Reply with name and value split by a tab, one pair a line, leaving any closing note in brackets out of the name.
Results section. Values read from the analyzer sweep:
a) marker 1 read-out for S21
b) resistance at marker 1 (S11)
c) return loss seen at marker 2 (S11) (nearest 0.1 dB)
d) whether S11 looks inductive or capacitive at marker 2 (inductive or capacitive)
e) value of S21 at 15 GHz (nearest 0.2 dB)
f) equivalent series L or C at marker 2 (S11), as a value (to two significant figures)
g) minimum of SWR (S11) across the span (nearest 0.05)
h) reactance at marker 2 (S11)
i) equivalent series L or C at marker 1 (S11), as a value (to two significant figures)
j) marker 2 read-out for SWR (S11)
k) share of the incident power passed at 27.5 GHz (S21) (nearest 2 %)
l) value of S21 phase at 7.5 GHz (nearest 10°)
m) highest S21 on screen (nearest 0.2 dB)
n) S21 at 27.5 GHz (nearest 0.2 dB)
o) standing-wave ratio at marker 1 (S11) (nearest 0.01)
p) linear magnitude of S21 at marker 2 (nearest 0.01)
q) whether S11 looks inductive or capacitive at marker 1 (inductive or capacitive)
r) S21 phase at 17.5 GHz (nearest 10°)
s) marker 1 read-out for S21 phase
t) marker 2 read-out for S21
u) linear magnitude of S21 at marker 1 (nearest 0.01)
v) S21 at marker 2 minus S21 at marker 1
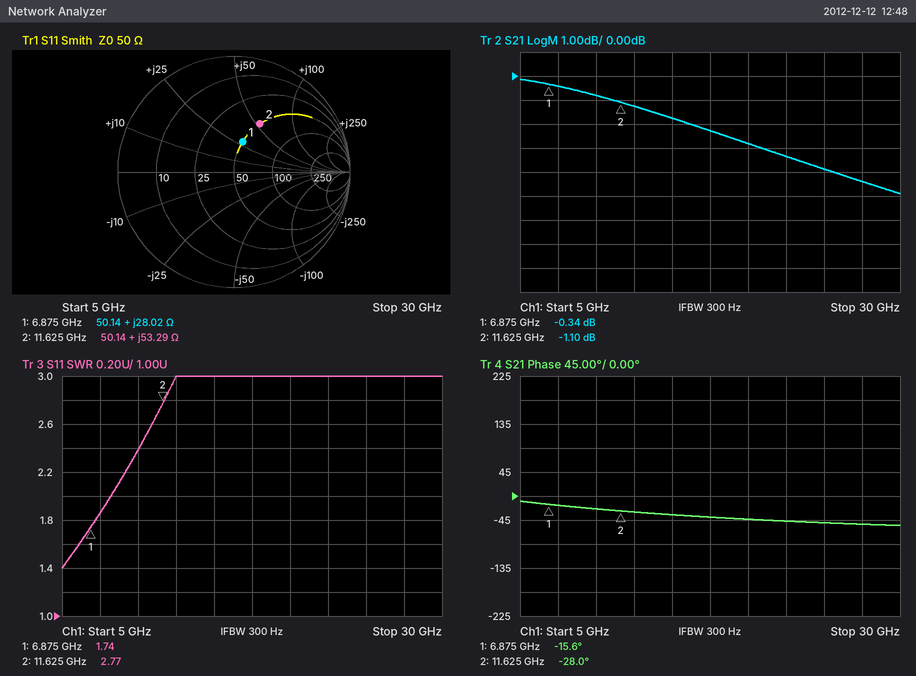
marker 1 read-out for S21	-0.34 dB
resistance at marker 1	50.14 Ω
return loss seen at marker 2 (S11)	6.6 dB
whether S11 looks inductive or capacitive at marker 2	inductive
value of S21 at 15 GHz	-1.8 dB
equivalent series L or C at marker 2 (S11), as a value	730 pH
minimum of SWR (S11) across the span	1.40
reactance at marker 2	+53.29 Ω
equivalent series L or C at marker 1 (S11), as a value	650 pH
marker 2 read-out for SWR	2.77
share of the incident power passed at 27.5 GHz (S21)	36 %
value of S21 phase at 7.5 GHz	-20°
highest S21 on screen	-0.2 dB
S21 at 27.5 GHz	-4.4 dB
standing-wave ratio at marker 1 (S11)	1.74
linear magnitude of S21 at marker 2	0.88
whether S11 looks inductive or capacitive at marker 1	inductive
S21 phase at 17.5 GHz	-40°
marker 1 read-out for S21 phase	-15.6°
marker 2 read-out for S21	-1.10 dB
linear magnitude of S21 at marker 1	0.96
S21 at marker 2 minus S21 at marker 1	-0.76 dB
